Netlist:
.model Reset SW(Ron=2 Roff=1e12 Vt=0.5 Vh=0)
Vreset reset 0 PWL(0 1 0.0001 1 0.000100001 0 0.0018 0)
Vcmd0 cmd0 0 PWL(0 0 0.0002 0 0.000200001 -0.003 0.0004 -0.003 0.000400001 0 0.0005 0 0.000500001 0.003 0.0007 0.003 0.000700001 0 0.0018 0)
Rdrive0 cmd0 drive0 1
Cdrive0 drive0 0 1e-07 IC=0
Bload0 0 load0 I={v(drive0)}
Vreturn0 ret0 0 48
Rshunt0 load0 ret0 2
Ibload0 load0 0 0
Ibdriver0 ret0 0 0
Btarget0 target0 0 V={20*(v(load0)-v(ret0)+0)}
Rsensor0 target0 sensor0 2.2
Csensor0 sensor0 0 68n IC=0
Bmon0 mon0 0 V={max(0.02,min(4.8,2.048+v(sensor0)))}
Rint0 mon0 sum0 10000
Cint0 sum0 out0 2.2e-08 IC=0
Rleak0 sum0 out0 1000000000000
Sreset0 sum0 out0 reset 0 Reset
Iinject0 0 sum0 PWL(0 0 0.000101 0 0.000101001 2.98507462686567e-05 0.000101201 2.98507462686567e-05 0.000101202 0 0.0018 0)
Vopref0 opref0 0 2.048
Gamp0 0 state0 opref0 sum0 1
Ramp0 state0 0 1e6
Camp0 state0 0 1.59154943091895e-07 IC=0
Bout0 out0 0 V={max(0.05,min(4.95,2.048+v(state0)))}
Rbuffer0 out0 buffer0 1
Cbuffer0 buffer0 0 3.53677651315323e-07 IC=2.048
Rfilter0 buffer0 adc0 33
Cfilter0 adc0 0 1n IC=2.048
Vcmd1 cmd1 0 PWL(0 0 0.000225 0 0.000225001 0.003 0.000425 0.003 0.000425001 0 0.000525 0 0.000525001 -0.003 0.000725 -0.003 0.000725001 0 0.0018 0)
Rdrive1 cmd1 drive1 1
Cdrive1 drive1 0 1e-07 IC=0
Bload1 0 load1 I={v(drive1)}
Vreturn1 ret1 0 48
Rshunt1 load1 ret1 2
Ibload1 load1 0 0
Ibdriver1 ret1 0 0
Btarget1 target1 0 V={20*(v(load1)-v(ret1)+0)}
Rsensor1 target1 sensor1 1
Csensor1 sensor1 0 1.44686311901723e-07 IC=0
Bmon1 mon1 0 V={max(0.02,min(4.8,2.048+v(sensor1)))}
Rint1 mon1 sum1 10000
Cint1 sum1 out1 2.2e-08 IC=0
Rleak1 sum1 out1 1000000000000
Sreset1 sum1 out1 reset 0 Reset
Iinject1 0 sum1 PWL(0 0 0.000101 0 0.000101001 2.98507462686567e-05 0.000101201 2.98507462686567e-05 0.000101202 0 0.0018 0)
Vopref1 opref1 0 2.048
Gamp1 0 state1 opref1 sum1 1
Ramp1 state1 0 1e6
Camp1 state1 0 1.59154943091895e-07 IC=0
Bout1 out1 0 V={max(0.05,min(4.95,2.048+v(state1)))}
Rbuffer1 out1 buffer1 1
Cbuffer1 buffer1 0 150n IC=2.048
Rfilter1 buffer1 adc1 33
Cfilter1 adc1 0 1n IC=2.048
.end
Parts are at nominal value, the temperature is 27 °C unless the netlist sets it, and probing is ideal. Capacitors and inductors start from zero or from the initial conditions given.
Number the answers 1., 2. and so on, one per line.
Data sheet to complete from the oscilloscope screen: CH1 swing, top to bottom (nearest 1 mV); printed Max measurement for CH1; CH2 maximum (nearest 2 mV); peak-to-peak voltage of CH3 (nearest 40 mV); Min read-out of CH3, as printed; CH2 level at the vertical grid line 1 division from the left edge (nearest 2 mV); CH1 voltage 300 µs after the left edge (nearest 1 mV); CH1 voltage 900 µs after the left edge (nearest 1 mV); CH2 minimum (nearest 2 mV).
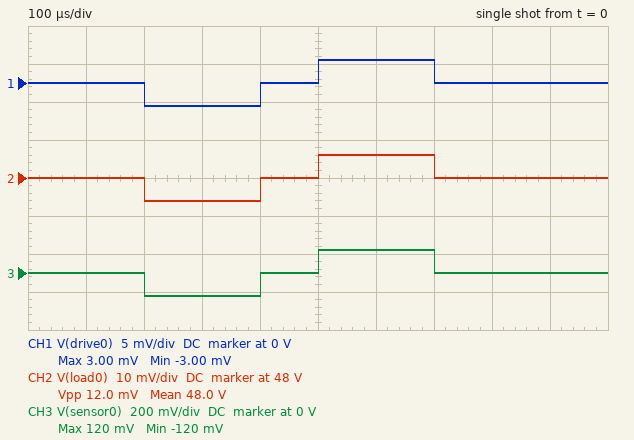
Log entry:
1. 6 mV
2. 3.00 mV
3. 48.006 V
4. 240 mV
5. -120 mV
6. 48.000 V
7. -3 mV
8. 0 V
9. 47.994 V
